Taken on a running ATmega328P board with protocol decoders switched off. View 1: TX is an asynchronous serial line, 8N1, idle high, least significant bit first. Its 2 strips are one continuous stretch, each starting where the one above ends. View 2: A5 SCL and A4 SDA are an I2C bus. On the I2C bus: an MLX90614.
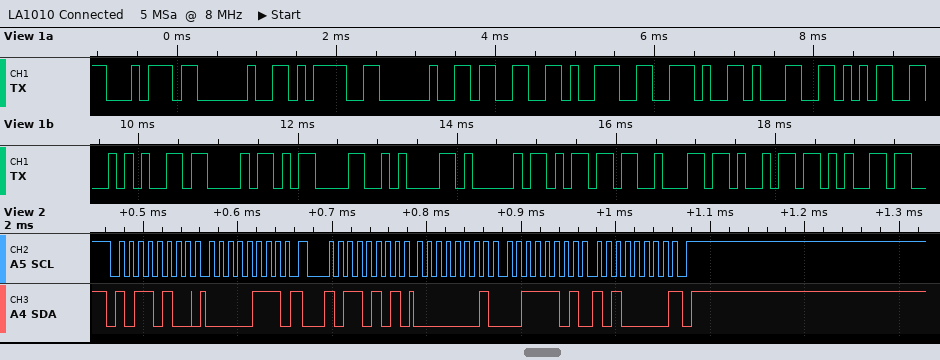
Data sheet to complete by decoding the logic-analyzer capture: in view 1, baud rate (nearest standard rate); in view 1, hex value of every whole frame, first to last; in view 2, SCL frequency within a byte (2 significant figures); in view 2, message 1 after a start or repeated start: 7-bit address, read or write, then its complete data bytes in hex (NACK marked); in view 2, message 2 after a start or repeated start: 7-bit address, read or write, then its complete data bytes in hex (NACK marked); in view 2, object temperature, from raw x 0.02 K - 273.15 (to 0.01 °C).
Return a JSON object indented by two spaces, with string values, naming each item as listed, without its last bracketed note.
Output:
{
  "in view 1, baud rate": "9600 baud",
  "in view 1, hex value of every whole frame, first to last": "74 20 3D 20 33 39 2E 31 35 2A 43 0D 0A 41 6D 62 69 65",
  "in view 2, SCL frequency within a byte": "100 kHz",
  "in view 2, message 1 after a start or repeated start: 7-bit address, read or write, then its complete data bytes in hex": "0x5A write: 07",
  "in view 2, message 2 after a start or repeated start: 7-bit address, read or write, then its complete data bytes in hex": "0x5A read: 01 3D A0 NACK",
  "in view 2, object temperature, from raw x 0.02 K - 273.15": "39.19 °C"
}
